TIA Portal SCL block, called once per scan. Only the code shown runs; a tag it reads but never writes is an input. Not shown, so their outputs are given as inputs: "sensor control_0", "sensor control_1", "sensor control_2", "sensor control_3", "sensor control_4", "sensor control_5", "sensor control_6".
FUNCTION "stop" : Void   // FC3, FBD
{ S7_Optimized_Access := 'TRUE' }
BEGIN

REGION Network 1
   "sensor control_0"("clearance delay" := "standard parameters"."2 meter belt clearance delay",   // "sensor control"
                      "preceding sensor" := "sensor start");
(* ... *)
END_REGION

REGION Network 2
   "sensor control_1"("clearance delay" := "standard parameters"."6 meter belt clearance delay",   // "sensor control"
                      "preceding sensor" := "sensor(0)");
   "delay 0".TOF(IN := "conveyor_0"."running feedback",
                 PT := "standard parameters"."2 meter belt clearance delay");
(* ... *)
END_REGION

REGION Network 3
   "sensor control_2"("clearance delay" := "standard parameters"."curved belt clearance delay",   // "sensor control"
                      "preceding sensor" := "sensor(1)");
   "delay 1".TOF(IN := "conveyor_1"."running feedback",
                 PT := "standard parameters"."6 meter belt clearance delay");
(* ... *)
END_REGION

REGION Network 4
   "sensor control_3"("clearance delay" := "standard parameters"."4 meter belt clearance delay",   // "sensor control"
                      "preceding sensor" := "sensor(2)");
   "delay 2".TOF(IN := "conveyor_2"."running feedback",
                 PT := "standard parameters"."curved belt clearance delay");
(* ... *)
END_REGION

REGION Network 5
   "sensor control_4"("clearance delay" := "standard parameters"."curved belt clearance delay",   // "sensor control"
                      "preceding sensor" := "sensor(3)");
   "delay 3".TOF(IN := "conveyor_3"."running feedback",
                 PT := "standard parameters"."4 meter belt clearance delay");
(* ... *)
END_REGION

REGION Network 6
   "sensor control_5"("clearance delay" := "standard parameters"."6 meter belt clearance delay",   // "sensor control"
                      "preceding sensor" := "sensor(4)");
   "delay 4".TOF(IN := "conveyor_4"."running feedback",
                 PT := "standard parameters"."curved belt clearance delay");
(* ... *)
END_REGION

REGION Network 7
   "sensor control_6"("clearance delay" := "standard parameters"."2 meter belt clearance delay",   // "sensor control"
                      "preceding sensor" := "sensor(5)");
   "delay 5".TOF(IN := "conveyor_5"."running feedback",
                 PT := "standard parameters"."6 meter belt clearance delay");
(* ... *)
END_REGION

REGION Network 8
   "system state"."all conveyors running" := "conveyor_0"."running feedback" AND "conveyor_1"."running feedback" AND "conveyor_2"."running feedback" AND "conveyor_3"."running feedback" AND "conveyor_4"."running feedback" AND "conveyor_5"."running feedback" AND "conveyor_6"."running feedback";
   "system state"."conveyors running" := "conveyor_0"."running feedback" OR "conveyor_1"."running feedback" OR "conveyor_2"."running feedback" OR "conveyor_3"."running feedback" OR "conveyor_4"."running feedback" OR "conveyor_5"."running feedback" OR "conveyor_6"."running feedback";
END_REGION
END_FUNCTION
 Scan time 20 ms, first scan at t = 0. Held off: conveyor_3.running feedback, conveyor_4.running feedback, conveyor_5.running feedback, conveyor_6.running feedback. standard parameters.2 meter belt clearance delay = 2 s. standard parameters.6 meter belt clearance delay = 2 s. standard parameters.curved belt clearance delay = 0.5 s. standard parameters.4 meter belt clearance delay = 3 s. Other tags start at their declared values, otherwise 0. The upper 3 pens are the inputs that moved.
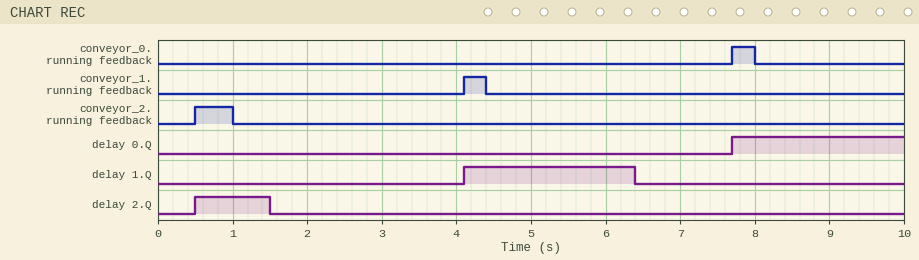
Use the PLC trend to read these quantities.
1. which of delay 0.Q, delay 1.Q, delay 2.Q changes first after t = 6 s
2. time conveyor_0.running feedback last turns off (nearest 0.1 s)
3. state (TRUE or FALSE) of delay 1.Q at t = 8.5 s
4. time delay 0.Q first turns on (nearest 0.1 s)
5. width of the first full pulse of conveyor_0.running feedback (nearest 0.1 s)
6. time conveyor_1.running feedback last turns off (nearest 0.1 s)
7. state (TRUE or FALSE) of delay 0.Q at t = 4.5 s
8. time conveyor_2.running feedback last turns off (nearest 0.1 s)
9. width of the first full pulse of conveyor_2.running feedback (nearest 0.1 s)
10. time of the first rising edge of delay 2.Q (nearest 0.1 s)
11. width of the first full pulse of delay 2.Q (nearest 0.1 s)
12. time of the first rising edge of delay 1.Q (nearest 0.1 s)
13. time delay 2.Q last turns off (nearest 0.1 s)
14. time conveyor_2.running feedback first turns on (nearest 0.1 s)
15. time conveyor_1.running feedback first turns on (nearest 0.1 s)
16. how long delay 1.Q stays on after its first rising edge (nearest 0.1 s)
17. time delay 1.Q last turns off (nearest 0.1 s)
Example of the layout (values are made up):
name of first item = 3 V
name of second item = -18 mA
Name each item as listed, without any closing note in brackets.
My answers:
which of delay 0.Q, delay 1.Q, delay 2.Q changes first after t = 6 s = delay 1.Q
time conveyor_0.running feedback last turns off = 8.0 s
state (TRUE or FALSE) of delay 1.Q at t = 8.5 s = FALSE
time delay 0.Q first turns on = 7.7 s
width of the first full pulse of conveyor_0.running feedback = 0.3 s
time conveyor_1.running feedback last turns off = 4.4 s
state (TRUE or FALSE) of delay 0.Q at t = 4.5 s = FALSE
time conveyor_2.running feedback last turns off = 1.0 s
width of the first full pulse of conveyor_2.running feedback = 0.5 s
time of the first rising edge of delay 2.Q = 0.5 s
width of the first full pulse of delay 2.Q = 1.0 s
time of the first rising edge of delay 1.Q = 4.1 s
time delay 2.Q last turns off = 1.5 s
time conveyor_2.running feedback first turns on = 0.5 s
time conveyor_1.running feedback first turns on = 4.1 s
how long delay 1.Q stays on after its first rising edge = 2.3 s
time delay 1.Q last turns off = 6.4 s
